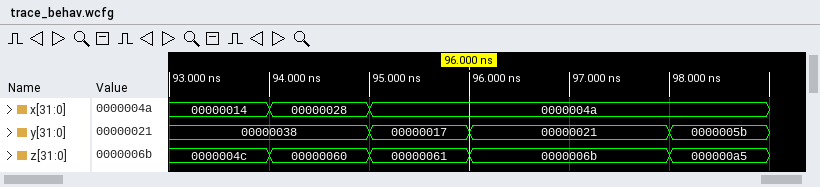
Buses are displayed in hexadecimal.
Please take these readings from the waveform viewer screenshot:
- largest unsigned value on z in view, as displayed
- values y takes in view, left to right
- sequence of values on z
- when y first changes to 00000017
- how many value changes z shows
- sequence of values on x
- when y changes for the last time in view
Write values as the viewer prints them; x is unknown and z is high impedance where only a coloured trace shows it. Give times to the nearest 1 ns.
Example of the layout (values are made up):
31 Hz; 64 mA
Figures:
000000a5; 00000038, 00000017, 00000021, 0000005b; 0000004c, 00000060, 00000061, 0000006b, 000000a5; 95 ns; 4; 00000014, 00000028, 0000004a; 98 ns
